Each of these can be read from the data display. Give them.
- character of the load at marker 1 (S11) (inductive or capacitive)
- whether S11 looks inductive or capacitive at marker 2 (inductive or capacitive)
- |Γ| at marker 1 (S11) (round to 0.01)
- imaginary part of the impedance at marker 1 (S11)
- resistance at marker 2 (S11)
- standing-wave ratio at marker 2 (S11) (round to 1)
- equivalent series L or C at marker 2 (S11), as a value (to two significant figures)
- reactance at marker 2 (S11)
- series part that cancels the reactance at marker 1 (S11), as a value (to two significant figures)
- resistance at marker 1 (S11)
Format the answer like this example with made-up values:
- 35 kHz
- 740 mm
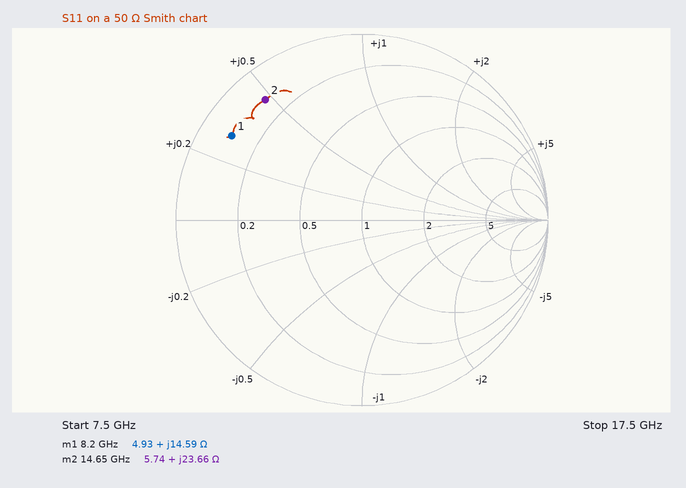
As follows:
- inductive
- inductive
- 0.83
- +14.59 Ω
- 5.74 Ω
- 11
- 260 pH
- +23.66 Ω
- 1.3 pF
- 4.93 Ω
